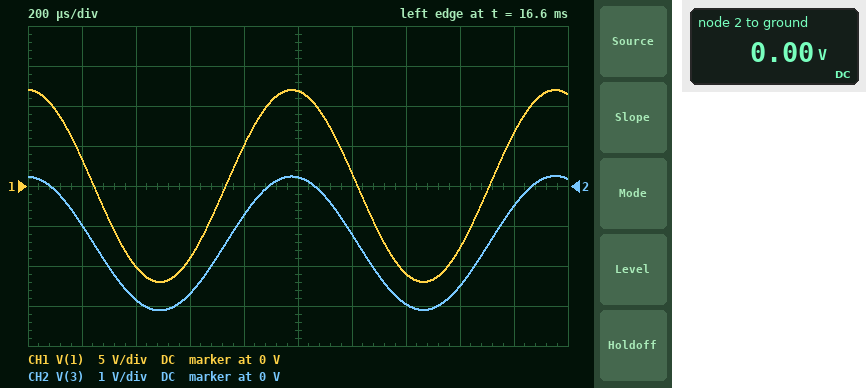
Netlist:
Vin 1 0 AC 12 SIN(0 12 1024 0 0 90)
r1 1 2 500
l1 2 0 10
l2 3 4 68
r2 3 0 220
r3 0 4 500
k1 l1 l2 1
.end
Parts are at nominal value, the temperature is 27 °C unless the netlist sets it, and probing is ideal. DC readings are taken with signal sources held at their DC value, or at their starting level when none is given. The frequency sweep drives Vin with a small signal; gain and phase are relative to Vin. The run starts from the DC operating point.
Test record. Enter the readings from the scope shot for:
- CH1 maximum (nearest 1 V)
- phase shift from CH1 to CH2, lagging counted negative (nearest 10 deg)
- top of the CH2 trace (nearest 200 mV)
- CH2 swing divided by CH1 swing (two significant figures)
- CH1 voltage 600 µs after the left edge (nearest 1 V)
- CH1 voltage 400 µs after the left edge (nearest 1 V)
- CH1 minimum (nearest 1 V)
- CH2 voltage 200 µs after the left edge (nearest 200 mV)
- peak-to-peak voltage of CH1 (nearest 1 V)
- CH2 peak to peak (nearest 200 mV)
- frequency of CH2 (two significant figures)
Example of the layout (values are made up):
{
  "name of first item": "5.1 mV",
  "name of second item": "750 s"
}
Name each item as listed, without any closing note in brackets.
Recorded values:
{
  "CH1 maximum": "12 V",
  "phase shift from CH1 to CH2, lagging counted negative": "0 deg",
  "top of the CH2 trace": "200 mV",
  "CH2 swing divided by CH1 swing": "0.14",
  "CH1 voltage 600 µs after the left edge": "-9 V",
  "CH1 voltage 400 µs after the left edge": "-10 V",
  "CH1 minimum": "-12 V",
  "CH2 voltage 200 µs after the left edge": "-1.0 V",
  "peak-to-peak voltage of CH1": "24 V",
  "CH2 peak to peak": "3.4 V",
  "frequency of CH2": "1.0 kHz"
}
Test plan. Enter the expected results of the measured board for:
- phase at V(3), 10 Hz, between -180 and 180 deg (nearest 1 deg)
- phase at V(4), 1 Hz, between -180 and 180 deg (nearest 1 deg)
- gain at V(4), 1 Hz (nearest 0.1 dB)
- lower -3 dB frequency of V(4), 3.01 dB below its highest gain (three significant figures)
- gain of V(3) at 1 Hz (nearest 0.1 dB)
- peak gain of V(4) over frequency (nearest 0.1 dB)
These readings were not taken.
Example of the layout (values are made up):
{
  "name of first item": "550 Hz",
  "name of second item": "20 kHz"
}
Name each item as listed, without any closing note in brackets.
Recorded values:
{
  "phase at V(3), 10 Hz, between -180 and 180 deg": "8 deg",
  "phase at V(4), 1 Hz, between -180 and 180 deg": "-126 deg",
  "gain at V(4), 1 Hz": "-14.7 dB",
  "lower -3 dB frequency of V(4), 3.01 dB below its highest gain": "1.39 Hz",
  "gain of V(3) at 1 Hz": "-21.8 dB",
  "peak gain of V(4) over frequency": "-10.0 dB"
}
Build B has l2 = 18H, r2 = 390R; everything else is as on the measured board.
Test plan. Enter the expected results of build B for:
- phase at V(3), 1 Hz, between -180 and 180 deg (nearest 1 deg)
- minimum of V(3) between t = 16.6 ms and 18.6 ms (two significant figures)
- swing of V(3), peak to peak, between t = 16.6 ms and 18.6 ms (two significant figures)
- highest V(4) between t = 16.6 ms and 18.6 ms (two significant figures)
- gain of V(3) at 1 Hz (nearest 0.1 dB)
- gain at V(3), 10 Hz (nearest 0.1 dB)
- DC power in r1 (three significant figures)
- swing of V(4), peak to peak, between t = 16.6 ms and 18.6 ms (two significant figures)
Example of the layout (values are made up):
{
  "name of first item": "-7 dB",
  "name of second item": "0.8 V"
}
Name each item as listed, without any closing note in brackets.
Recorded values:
{
  "phase at V(3), 1 Hz, between -180 and 180 deg": "76 deg",
  "minimum of V(3) between t = 16.6 ms and 18.6 ms": "-5.8 V",
  "swing of V(3), peak to peak, between t = 16.6 ms and 18.6 ms": "7.1 V",
  "highest V(4) between t = 16.6 ms and 18.6 ms": "7.4 V",
  "gain of V(3) at 1 Hz": "-22.9 dB",
  "gain at V(3), 10 Hz": "-11.3 dB",
  "DC power in r1": "288 mW",
  "swing of V(4), peak to peak, between t = 16.6 ms and 18.6 ms": "9.1 V"
}
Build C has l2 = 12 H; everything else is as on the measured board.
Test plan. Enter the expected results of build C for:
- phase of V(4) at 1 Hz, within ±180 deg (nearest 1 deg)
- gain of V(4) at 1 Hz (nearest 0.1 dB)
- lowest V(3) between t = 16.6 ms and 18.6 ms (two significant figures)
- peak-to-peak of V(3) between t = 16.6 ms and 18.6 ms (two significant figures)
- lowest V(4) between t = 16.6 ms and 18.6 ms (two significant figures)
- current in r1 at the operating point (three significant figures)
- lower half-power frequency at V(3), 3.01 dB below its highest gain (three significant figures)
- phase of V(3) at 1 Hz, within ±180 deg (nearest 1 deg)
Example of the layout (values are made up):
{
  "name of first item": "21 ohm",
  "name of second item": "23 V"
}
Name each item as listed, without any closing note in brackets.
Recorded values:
{
  "phase of V(4) at 1 Hz, within ±180 deg": "-103 deg",
  "gain of V(4) at 1 Hz": "-20.6 dB",
  "lowest V(3) between t = 16.6 ms and 18.6 ms": "-3.6 V",
  "peak-to-peak of V(3) between t = 16.6 ms and 18.6 ms": "4.4 V",
  "lowest V(4) between t = 16.6 ms and 18.6 ms": "-2.0 V",
  "current in r1 at the operating point": "24.0 mA",
  "lower half-power frequency at V(3), 3.01 dB below its highest gain": "4.34 Hz",
  "phase of V(3) at 1 Hz, within ±180 deg": "77 deg"
}
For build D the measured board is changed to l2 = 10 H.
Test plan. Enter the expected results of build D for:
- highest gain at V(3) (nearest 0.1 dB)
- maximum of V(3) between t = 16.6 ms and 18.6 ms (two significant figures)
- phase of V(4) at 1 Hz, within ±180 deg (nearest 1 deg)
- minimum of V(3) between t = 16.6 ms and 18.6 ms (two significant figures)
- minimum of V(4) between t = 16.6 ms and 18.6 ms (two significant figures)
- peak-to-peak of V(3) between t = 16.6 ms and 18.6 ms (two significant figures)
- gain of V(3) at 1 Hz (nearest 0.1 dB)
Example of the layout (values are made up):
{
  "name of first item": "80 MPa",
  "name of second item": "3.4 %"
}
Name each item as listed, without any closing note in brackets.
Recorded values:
{
  "highest gain at V(3)": "-14.9 dB",
  "maximum of V(3) between t = 16.6 ms and 18.6 ms": "910 mV",
  "phase of V(4) at 1 Hz, within ±180 deg": "-102 deg",
  "minimum of V(3) between t = 16.6 ms and 18.6 ms": "-3.5 V",
  "minimum of V(4) between t = 16.6 ms and 18.6 ms": "-2.1 V",
  "peak-to-peak of V(3) between t = 16.6 ms and 18.6 ms": "4.4 V",
  "gain of V(3) at 1 Hz": "-28.5 dB"
}
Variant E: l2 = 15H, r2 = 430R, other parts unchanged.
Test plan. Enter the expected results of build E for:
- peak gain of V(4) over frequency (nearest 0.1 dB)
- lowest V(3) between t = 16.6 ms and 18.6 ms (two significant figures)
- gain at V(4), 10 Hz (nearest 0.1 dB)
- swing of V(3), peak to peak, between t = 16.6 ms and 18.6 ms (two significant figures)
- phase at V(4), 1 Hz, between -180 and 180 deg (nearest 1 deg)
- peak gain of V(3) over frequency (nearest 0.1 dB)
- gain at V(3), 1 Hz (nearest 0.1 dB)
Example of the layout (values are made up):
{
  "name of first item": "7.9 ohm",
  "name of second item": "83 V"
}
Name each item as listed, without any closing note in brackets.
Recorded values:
{
  "peak gain of V(4) over frequency": "-8.8 dB",
  "lowest V(3) between t = 16.6 ms and 18.6 ms": "-6.1 V",
  "gain at V(4), 10 Hz": "-9.5 dB",
  "swing of V(3), peak to peak, between t = 16.6 ms and 18.6 ms": "7.6 V",
  "phase at V(4), 1 Hz, between -180 and 180 deg": "-103 deg",
  "peak gain of V(3) over frequency": "-10.1 dB",
  "gain at V(3), 1 Hz": "-23.2 dB"
}
